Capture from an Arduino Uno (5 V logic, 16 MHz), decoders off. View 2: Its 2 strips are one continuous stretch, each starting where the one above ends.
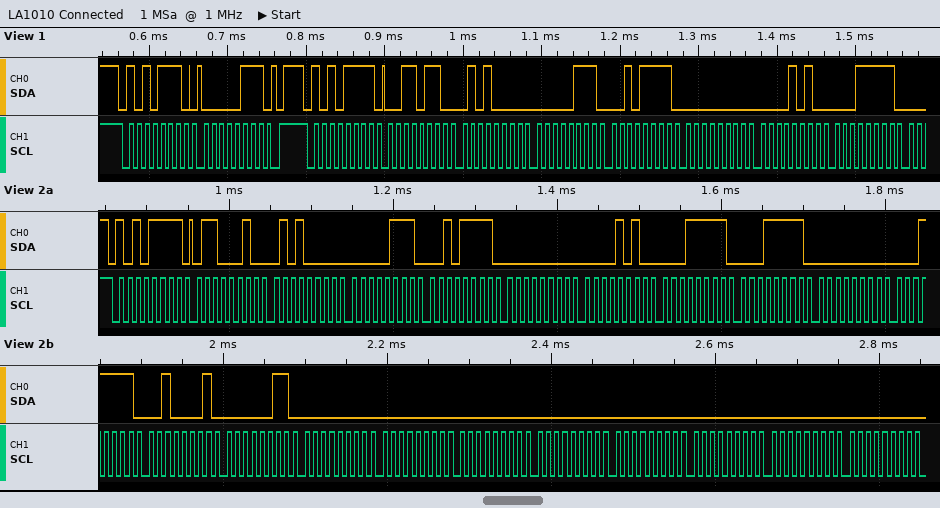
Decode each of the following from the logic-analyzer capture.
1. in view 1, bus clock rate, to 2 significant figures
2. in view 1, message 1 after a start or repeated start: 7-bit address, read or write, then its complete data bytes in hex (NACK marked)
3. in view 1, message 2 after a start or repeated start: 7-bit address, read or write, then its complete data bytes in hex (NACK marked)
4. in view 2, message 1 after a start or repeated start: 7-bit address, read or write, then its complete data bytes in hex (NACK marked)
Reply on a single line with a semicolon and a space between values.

100 kHz; 0x57 write: 07; 0x57 read: 36 50 07 2F 00 0A 1F; 0x57 read: 62 50 07 2F 00 0A 1F 1F 00 1F 21 03 00 00 00 00 00 00 00 00
